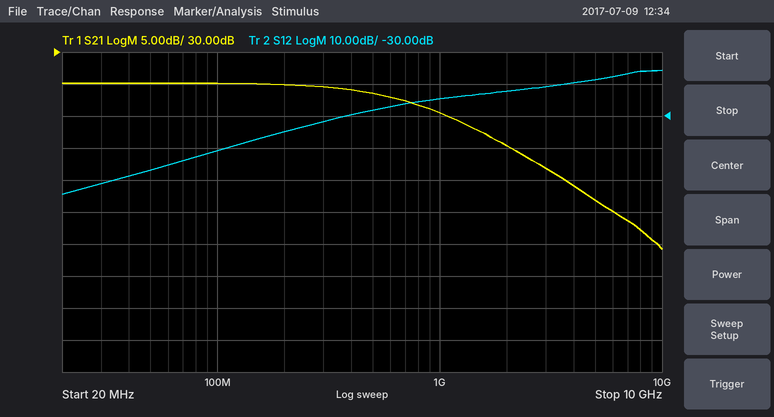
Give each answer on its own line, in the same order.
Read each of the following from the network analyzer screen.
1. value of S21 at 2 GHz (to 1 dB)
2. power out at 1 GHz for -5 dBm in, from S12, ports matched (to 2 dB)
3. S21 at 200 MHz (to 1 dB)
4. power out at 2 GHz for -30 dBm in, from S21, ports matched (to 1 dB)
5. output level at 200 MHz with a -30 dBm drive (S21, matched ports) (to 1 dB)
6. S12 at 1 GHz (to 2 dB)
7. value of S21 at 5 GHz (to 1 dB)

15 dB
-30 dBm
25 dB
-15 dBm
-5 dBm
-24 dB
7 dB
